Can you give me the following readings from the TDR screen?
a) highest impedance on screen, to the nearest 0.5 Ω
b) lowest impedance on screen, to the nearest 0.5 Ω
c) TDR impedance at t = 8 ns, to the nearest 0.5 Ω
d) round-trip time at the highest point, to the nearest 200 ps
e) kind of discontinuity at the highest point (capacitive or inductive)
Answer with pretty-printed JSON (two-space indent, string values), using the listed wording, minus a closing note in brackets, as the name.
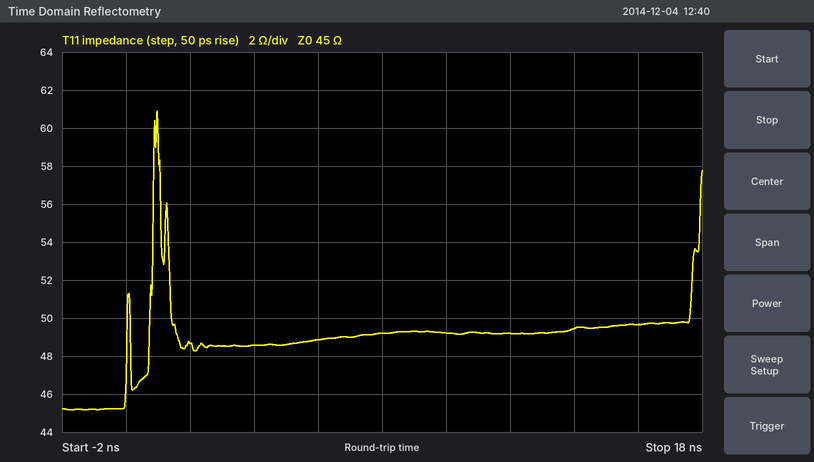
{
  "highest impedance on screen, to the nearest 0.5 Ω": "61.0 Ω",
  "lowest impedance on screen, to the nearest 0.5 Ω": "45.0 Ω",
  "TDR impedance at t = 8 ns, to the nearest 0.5 Ω": "49.0 Ω",
  "round-trip time at the highest point, to the nearest 200 ps": "1.0 ns",
  "kind of discontinuity at the highest point": "inductive"
}
